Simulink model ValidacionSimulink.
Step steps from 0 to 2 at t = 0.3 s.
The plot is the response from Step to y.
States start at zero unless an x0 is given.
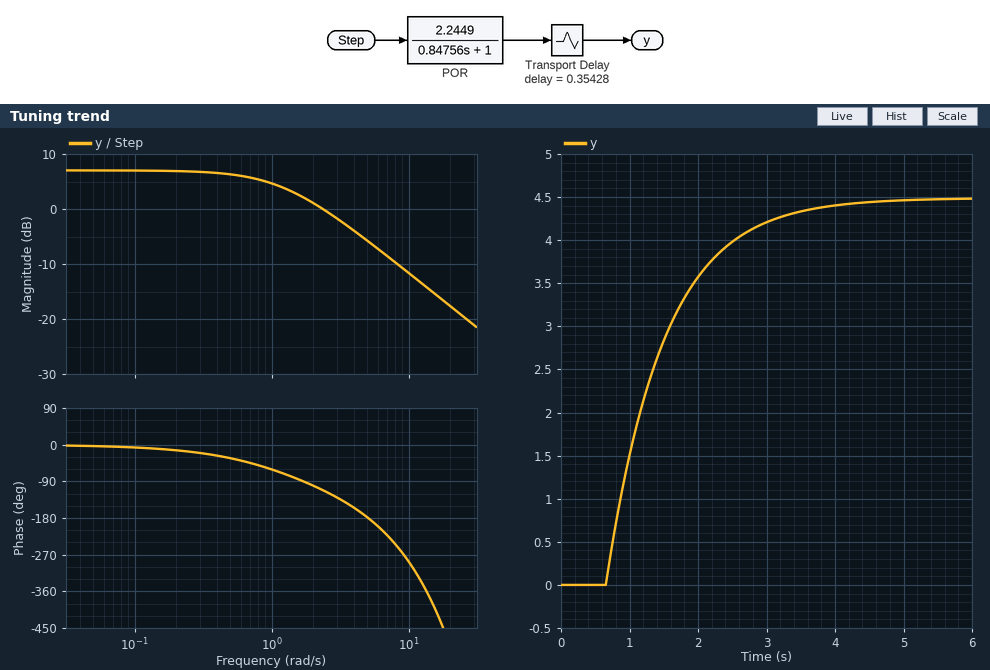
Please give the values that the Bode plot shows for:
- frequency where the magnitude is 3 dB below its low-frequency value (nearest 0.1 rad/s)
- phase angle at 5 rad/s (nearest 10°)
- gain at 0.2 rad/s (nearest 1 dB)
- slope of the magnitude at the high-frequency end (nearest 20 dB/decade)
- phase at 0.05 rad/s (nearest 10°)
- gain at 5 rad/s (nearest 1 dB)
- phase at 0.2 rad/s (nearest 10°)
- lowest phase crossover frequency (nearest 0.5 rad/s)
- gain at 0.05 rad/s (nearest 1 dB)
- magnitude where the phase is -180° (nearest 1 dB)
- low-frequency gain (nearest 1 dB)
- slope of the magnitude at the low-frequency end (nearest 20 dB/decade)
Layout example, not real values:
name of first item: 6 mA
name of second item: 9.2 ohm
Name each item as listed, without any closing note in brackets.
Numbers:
frequency where the magnitude is 3 dB below its low-frequency value: 1.2 rad/s
phase angle at 5 rad/s: -180°
gain at 0.2 rad/s: 7 dB
slope of the magnitude at the high-frequency end: -20 dB/decade
phase at 0.05 rad/s: 0°
gain at 5 rad/s: -6 dB
phase at 0.2 rad/s: -10°
lowest phase crossover frequency: 5.0 rad/s
gain at 0.05 rad/s: 7 dB
magnitude where the phase is -180°: -6 dB
low-frequency gain: 7 dB
slope of the magnitude at the low-frequency end: 0 dB/decade
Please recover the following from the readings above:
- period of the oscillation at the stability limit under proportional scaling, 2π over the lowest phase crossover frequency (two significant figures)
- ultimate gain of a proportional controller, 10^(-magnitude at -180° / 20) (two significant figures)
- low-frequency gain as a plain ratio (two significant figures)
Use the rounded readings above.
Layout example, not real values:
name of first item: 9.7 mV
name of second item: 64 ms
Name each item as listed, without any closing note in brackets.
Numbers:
period of the oscillation at the stability limit under proportional scaling, 2π over the lowest phase crossover frequency: 1.3 s
ultimate gain of a proportional controller, 10^(-magnitude at -180° / 20): 2.0
low-frequency gain as a plain ratio: 2.2
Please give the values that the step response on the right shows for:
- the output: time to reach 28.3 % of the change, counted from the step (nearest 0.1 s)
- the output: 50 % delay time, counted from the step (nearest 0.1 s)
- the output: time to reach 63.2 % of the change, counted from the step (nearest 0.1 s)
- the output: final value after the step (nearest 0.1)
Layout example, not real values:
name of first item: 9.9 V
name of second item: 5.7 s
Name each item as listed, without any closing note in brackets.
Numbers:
the output: time to reach 28.3 % of the change, counted from the step: 0.6 s
the output: 50 % delay time, counted from the step: 0.9 s
the output: time to reach 63.2 % of the change, counted from the step: 1.2 s
the output: final value after the step: 4.5
